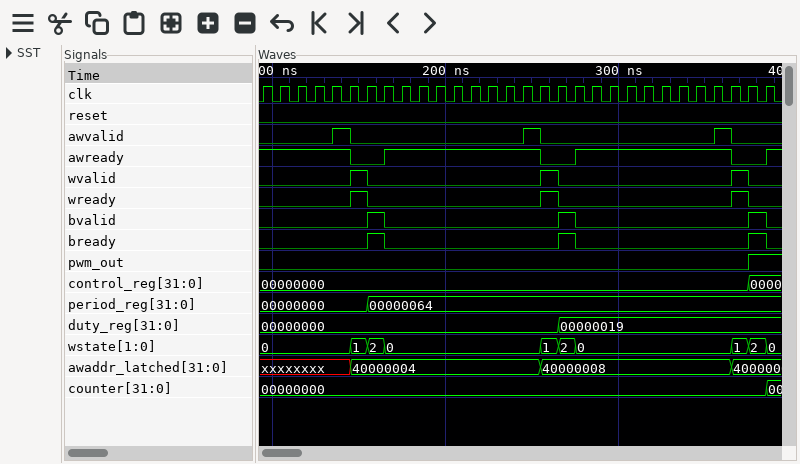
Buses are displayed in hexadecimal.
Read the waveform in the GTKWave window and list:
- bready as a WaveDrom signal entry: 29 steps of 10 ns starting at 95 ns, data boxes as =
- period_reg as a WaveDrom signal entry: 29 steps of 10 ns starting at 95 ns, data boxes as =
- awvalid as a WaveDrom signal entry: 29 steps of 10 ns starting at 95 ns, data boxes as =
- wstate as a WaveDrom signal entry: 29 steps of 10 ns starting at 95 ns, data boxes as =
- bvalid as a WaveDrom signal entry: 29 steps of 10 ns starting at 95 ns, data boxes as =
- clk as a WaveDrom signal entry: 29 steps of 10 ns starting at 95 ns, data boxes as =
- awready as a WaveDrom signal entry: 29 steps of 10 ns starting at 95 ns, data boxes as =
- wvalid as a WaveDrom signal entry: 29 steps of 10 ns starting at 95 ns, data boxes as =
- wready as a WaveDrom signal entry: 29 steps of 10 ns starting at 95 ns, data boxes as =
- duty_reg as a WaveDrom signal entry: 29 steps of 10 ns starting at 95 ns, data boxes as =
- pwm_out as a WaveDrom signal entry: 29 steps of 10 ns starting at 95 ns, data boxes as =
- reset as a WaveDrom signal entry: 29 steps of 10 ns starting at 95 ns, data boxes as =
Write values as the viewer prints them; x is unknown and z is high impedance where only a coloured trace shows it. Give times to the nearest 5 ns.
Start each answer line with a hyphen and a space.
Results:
- {name: 'bready', wave: '0.....10.........10.........1'}
- {name: 'period_reg', wave: '=.....=......................', data: '00000000 00000064'}
- {name: 'awvalid', wave: '0...10.........10.........10.'}
- {name: 'wstate', wave: '=....===........===........==', data: '0 1 2 0 1 2 0 1 2'}
- {name: 'bvalid', wave: '0.....10.........10.........1'}
- {name: 'clk', wave: 'p............................'}
- {name: 'awready', wave: '1....0.1........0.1........0.'}
- {name: 'wvalid', wave: '0....10.........10.........10'}
- {name: 'wready', wave: '0....10.........10.........10'}
- {name: 'duty_reg', wave: '=................=...........', data: '00000000 00000019'}
- {name: 'pwm_out', wave: '0...........................1'}
- {name: 'reset', wave: '0............................'}
